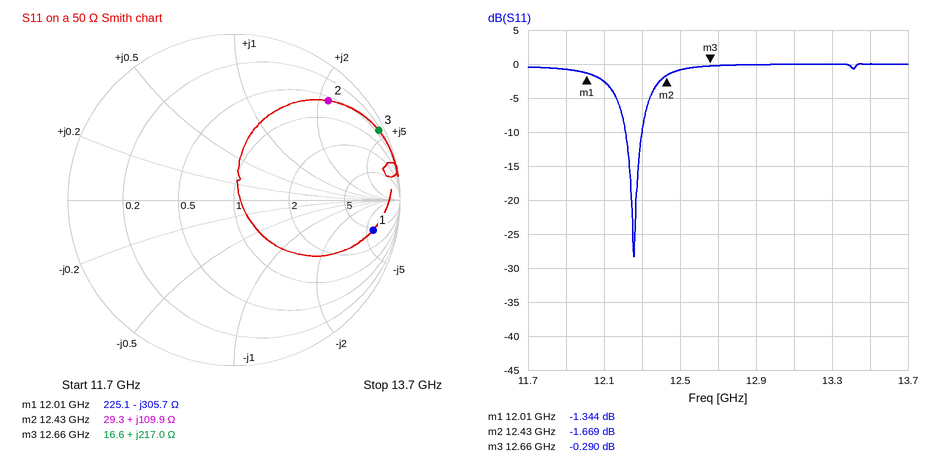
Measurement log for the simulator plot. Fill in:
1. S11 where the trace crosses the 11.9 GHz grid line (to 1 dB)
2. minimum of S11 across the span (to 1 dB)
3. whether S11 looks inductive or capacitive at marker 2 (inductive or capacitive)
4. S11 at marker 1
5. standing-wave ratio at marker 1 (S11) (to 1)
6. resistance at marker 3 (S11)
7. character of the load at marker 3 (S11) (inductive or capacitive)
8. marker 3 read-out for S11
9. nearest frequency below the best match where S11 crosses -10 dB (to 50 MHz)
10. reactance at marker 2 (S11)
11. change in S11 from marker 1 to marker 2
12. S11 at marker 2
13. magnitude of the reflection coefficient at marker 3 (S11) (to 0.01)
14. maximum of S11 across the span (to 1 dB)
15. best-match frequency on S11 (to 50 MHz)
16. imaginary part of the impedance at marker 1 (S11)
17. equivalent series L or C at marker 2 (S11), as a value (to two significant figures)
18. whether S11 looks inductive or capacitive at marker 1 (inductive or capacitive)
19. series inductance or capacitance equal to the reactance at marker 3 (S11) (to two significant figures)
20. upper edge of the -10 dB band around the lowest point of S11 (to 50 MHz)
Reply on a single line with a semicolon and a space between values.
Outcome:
-1 dB; -28 dB; inductive; -1.344 dB; 13; 16.6 Ω; inductive; -0.290 dB; 12.20 GHz; +109.9 Ω; -0.325 dB; -1.669 dB; 0.97; 0 dB; 12.25 GHz; -305.7 Ω; 1.4 nH; capacitive; 2.7 nH; 12.30 GHz
